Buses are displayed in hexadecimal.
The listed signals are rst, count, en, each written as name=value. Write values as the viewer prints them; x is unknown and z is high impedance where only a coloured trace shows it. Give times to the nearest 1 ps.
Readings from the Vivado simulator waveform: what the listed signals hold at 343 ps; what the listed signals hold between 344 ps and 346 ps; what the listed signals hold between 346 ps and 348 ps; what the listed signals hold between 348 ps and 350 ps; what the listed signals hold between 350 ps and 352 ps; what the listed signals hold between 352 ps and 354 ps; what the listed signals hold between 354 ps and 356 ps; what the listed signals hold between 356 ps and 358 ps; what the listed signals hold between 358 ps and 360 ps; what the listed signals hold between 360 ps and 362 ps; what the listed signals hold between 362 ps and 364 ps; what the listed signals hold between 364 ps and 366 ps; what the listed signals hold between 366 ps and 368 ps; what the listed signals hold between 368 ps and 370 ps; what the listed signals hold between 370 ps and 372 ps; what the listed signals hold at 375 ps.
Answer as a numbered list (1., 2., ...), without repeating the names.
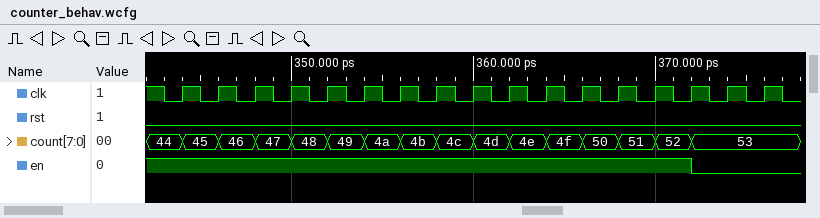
1. rst=0, count=44, en=1
2. rst=0, count=45, en=1
3. rst=0, count=46, en=1
4. rst=0, count=47, en=1
5. rst=0, count=48, en=1
6. rst=0, count=49, en=1
7. rst=0, count=4a, en=1
8. rst=0, count=4b, en=1
9. rst=0, count=4c, en=1
10. rst=0, count=4d, en=1
11. rst=0, count=4e, en=1
12. rst=0, count=4f, en=1
13. rst=0, count=50, en=1
14. rst=0, count=51, en=1
15. rst=0, count=52, en=1
16. rst=0, count=53, en=0
